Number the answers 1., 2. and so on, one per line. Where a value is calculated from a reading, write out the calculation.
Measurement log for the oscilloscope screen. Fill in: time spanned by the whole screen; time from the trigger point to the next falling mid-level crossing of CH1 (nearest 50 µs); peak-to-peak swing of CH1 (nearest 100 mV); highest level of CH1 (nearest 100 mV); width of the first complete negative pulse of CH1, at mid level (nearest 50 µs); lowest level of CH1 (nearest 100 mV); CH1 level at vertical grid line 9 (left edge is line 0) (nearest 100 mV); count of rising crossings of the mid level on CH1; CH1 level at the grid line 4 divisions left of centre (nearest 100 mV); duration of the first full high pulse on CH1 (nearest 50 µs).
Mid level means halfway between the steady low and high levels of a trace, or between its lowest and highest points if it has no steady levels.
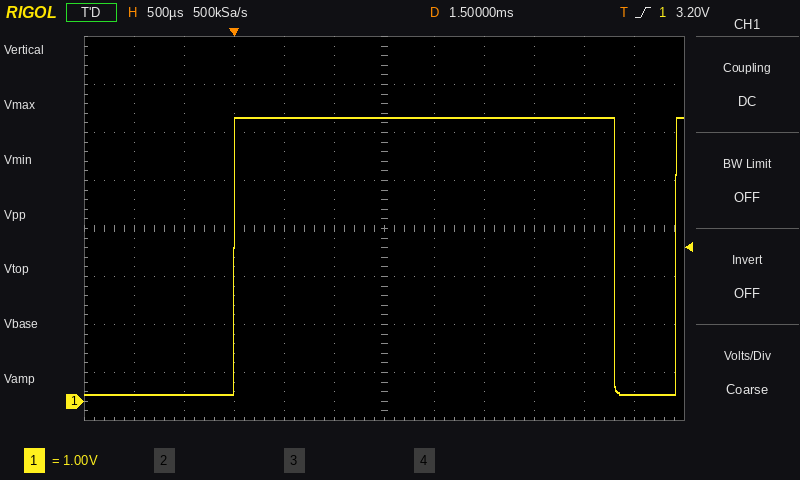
1. 6 ms
2. 3.80 ms
3. 5.9 V − (100 mV) = 5.8 V
4. 5.9 V
5. 600 µs
6. 100 mV
7. 5.9 V
8. 2
9. 100 mV
10. 3.80 ms
